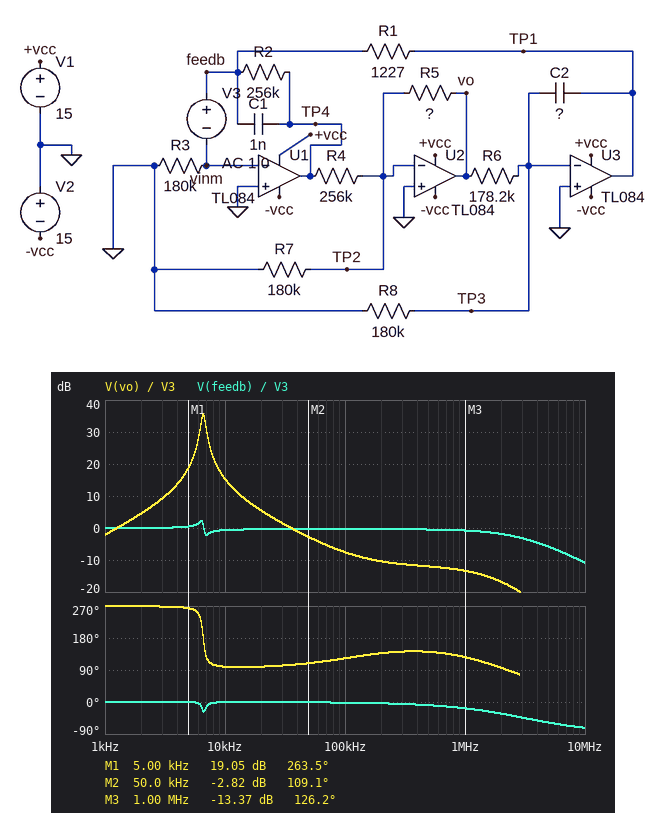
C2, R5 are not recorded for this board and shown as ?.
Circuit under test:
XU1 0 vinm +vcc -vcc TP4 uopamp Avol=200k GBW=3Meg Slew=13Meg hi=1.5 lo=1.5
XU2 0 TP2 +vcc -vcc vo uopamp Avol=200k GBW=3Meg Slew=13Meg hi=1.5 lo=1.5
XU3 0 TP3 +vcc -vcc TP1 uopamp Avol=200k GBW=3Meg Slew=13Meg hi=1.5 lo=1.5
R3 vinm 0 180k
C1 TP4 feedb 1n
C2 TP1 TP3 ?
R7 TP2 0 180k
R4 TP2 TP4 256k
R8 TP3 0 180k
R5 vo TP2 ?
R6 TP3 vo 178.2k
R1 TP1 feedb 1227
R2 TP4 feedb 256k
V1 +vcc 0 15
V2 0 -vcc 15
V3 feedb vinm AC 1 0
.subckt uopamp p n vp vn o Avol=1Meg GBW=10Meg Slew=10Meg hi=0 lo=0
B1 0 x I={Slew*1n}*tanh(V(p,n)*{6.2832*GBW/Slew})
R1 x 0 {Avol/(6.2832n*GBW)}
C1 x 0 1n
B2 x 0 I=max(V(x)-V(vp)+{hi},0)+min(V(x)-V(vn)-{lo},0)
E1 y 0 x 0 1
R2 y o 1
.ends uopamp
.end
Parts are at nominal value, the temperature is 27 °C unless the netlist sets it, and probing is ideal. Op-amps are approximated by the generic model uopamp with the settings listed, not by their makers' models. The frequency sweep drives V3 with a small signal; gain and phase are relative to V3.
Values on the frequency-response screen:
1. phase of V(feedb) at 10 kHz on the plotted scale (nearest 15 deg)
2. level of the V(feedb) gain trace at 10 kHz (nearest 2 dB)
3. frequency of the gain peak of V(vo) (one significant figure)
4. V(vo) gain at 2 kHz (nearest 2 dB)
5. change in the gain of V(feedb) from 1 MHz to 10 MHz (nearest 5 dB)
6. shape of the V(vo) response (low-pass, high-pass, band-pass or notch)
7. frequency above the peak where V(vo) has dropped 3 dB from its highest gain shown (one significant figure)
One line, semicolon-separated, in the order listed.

0 deg; 0 dB; 7 kHz; 4 dB; -10 dB; band-pass; 7 kHz
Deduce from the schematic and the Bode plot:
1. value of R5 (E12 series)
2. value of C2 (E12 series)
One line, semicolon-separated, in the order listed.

68 kΩ; 680 pF
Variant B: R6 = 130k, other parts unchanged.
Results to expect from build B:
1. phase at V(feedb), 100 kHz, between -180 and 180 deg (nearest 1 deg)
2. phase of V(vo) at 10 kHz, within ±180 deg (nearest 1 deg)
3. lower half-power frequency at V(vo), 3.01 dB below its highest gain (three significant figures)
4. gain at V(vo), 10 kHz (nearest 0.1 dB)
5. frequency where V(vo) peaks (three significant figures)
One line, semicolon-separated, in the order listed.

-2 deg; 101 deg; 7.45 kHz; 18.2 dB; 7.71 kHz
